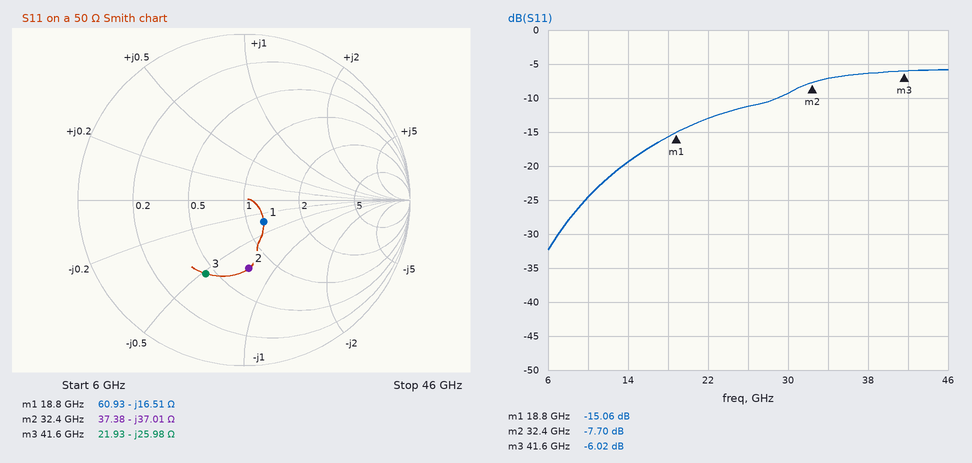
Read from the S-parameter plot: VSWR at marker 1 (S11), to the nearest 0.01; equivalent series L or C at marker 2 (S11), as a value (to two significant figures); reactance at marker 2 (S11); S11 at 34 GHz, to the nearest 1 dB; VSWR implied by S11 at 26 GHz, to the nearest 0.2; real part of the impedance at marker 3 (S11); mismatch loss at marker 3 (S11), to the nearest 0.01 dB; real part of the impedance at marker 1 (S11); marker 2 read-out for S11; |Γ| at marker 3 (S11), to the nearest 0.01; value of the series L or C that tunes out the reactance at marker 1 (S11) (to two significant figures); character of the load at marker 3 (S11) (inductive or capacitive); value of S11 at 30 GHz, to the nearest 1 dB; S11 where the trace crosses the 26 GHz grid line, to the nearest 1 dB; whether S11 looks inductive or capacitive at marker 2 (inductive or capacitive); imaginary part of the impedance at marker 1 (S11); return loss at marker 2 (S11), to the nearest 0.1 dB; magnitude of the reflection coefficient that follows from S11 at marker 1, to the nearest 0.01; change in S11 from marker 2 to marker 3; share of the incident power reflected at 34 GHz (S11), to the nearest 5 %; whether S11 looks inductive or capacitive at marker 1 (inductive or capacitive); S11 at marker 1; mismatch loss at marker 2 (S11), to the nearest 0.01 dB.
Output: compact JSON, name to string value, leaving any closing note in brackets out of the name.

{"VSWR at marker 1 (S11), to the nearest 0.01": "1.43", "equivalent series L or C at marker 2 (S11), as a value": "130 fF", "reactance at marker 2": "-37.01 Ω", "S11 at 34 GHz, to the nearest 1 dB": "-7 dB", "VSWR implied by S11 at 26 GHz, to the nearest 0.2": "1.8", "real part of the impedance at marker 3": "21.93 Ω", "mismatch loss at marker 3 (S11), to the nearest 0.01 dB": "1.25 dB", "real part of the impedance at marker 1": "60.93 Ω", "marker 2 read-out for S11": "-7.70 dB", "|Γ| at marker 3 (S11), to the nearest 0.01": "0.50", "value of the series L or C that tunes out the reactance at marker 1 (S11)": "140 pH", "character of the load at marker 3 (S11)": "capacitive", "value of S11 at 30 GHz, to the nearest 1 dB": "-9 dB", "S11 where the trace crosses the 26 GHz grid line, to the nearest 1 dB": "-11 dB", "whether S11 looks inductive or capacitive at marker 2": "capacitive", "imaginary part of the impedance at marker 1": "-16.51 Ω", "return loss at marker 2 (S11), to the nearest 0.1 dB": "7.7 dB", "magnitude of the reflection coefficient that follows from S11 at marker 1, to the nearest 0.01": "0.18", "change in S11 from marker 2 to marker 3": "1.68 dB", "share of the incident power reflected at 34 GHz (S11), to the nearest 5 %": "20 %", "whether S11 looks inductive or capacitive at marker 1": "capacitive", "S11 at marker 1": "-15.06 dB", "mismatch loss at marker 2 (S11), to the nearest 0.01 dB": "0.81 dB"}
